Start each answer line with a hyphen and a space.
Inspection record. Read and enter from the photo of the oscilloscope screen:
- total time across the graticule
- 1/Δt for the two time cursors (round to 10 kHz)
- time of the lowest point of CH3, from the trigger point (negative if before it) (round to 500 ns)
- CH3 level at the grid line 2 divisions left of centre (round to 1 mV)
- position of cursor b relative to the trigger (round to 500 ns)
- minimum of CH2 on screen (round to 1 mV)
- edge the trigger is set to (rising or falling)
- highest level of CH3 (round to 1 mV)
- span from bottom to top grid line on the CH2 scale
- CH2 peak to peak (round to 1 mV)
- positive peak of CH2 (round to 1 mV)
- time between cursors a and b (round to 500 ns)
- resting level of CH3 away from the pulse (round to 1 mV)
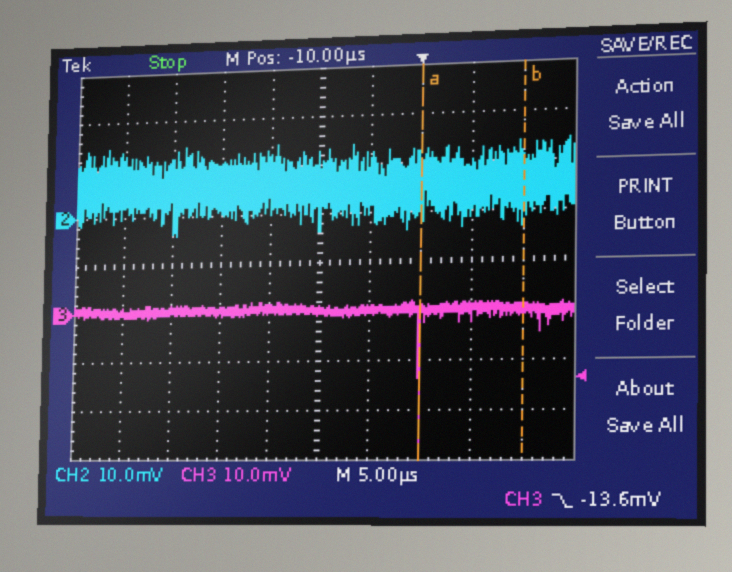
- 50 µs
- 100 kHz
- 0.0 µs
- 0 mV
- +10.0 µs
- -4 mV
- falling
- 2 mV
- 80 mV
- 18 mV
- 14 mV
- 10.0 µs
- 0 mV
